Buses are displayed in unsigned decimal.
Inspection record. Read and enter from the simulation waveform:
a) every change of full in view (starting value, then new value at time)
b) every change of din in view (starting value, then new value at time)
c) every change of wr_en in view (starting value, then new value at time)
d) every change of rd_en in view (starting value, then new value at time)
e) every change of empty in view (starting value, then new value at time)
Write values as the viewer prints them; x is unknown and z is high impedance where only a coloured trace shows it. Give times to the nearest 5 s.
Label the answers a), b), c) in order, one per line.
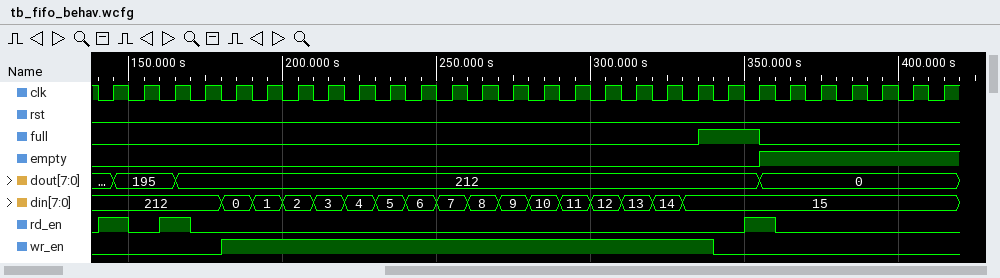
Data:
a) 0, 1 at 335 s, 0 at 355 s
b) 212, 0 at 180 s, 1 at 190 s, 2 at 200 s, 3 at 210 s, 4 at 220 s, 5 at 230 s, 6 at 240 s, 7 at 250 s, 8 at 260 s, 9 at 270 s, 10 at 280 s, 11 at 290 s, 12 at 300 s, 13 at 310 s, 14 at 320 s, 15 at 330 s
c) 0, 1 at 180 s, 0 at 340 s
d) 0, 1 at 140 s, 0 at 150 s, 1 at 160 s, 0 at 170 s, 1 at 350 s, 0 at 360 s
e) 0, 1 at 355 s
